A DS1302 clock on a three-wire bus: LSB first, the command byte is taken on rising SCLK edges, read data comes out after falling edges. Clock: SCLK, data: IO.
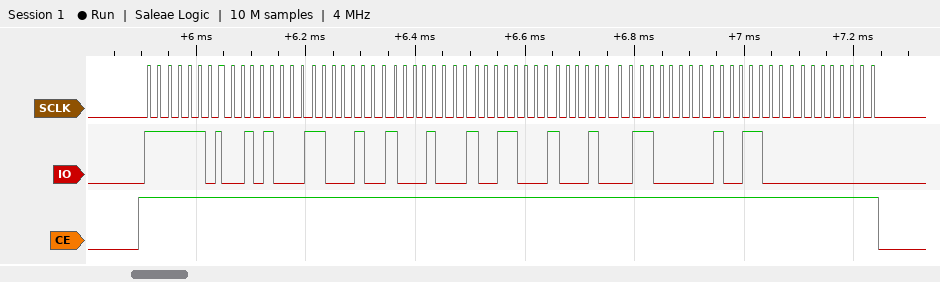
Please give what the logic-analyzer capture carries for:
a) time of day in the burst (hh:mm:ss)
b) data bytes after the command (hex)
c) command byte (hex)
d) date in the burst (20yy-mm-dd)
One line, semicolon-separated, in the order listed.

11:23:14; 14 23 11 19 11 03 19 00; 0xBF; 2019-11-19
